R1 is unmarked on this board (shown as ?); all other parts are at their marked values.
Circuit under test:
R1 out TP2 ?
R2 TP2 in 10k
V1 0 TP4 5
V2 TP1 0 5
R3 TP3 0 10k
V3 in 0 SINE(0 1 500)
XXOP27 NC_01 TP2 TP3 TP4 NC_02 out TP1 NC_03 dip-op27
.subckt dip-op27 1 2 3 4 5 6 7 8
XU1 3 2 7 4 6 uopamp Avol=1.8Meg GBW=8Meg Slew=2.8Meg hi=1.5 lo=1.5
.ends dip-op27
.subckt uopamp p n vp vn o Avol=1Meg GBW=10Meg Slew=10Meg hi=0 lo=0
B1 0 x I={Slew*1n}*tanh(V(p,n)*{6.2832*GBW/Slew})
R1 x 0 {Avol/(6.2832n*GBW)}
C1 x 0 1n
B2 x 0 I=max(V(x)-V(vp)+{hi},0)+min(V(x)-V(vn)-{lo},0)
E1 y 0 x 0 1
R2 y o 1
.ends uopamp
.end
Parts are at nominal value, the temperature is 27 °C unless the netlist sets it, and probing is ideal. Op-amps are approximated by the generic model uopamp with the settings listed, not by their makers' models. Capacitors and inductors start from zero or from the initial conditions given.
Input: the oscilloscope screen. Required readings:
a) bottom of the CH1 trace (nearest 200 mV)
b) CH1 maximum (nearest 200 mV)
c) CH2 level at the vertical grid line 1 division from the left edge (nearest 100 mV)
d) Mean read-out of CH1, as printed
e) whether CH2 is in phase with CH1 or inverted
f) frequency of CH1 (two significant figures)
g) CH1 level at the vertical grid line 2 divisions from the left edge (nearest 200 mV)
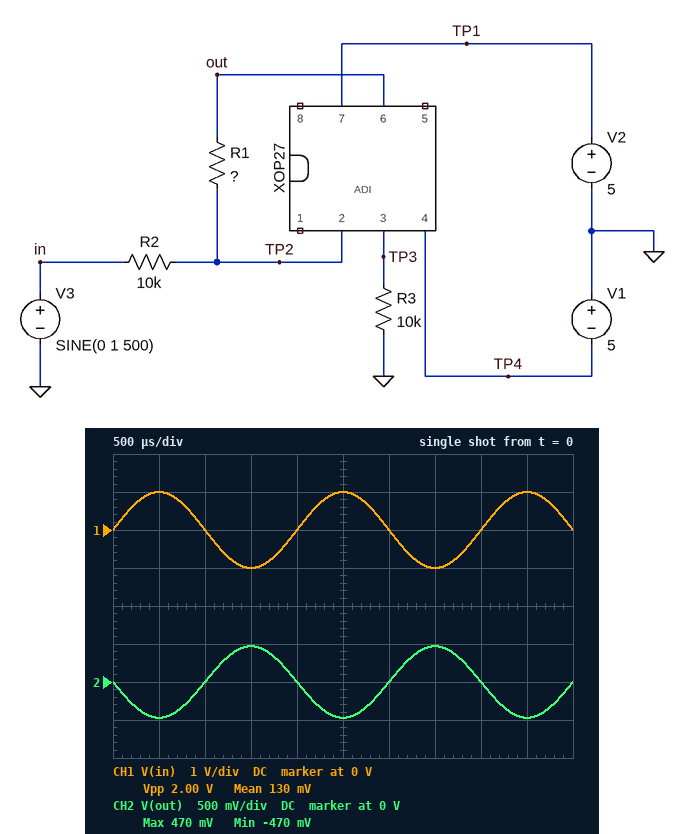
-1.0 V
1.0 V
-500 mV
130 mV
inverted
500 Hz
0 V
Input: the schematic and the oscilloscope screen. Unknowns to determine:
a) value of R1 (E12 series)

4.7 kΩ
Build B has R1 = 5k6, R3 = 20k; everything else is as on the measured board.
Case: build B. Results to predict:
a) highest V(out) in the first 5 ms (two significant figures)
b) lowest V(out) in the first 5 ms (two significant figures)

560 mV
-560 mV
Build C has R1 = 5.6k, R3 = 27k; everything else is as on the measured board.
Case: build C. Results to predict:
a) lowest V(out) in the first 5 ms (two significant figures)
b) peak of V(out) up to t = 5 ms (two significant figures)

-560 mV
560 mV
